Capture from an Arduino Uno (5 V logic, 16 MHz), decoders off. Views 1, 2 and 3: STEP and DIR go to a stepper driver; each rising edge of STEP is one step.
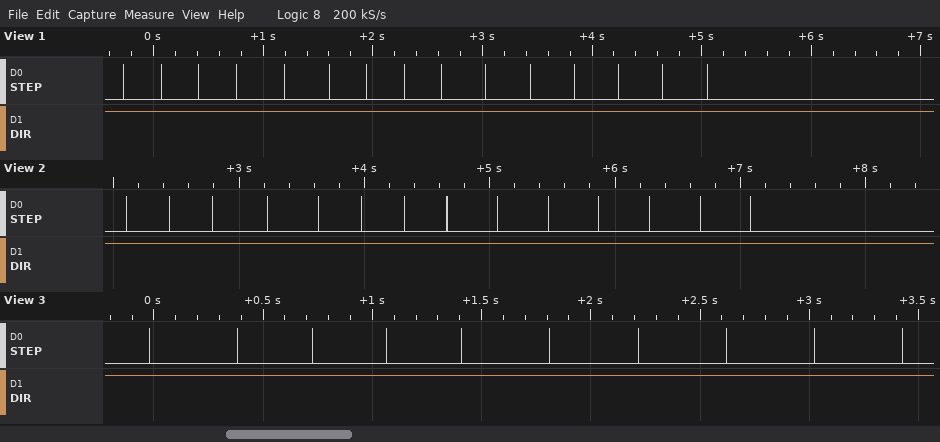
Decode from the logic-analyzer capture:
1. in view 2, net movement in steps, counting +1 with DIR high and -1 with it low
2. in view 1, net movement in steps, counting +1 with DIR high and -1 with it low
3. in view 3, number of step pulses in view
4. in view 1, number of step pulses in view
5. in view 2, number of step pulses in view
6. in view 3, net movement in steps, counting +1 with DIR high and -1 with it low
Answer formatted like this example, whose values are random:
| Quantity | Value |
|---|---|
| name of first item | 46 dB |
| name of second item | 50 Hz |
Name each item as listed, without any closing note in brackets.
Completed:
| Quantity | Value |
|---|---|
| in view 2, net movement in steps, counting +1 with DIR high and -1 with it low | +14 |
| in view 1, net movement in steps, counting +1 with DIR high and -1 with it low | +15 |
| in view 3, number of step pulses in view | 10 |
| in view 1, number of step pulses in view | 15 |
| in view 2, number of step pulses in view | 14 |
| in view 3, net movement in steps, counting +1 with DIR high and -1 with it low | +10 |
